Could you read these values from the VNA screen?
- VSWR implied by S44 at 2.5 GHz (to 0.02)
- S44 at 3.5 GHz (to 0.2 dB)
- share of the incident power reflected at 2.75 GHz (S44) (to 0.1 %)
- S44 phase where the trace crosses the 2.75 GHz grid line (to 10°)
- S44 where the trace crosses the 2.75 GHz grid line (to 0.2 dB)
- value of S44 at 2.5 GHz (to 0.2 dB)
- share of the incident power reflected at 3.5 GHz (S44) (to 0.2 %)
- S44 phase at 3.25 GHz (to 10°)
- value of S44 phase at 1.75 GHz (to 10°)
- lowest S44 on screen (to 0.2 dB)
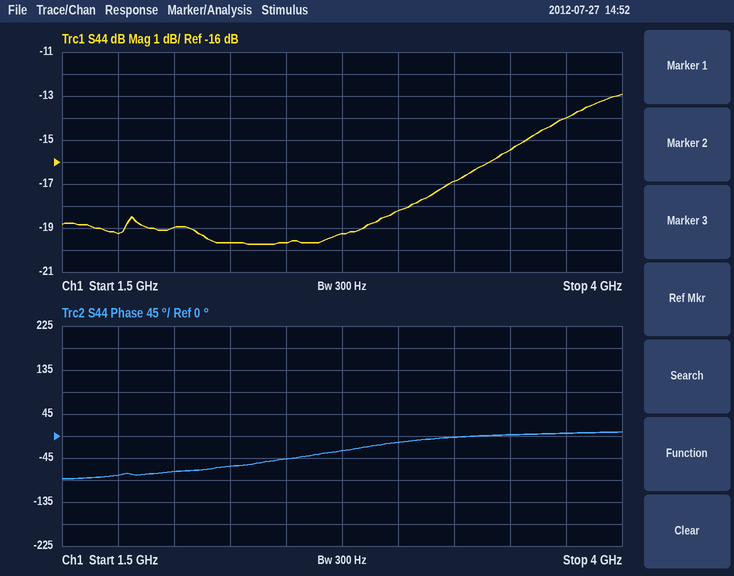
1.24
-15.4 dB
1.2 %
-30°
-19.2 dB
-19.6 dB
2.8 %
0°
-80°
-19.8 dB
